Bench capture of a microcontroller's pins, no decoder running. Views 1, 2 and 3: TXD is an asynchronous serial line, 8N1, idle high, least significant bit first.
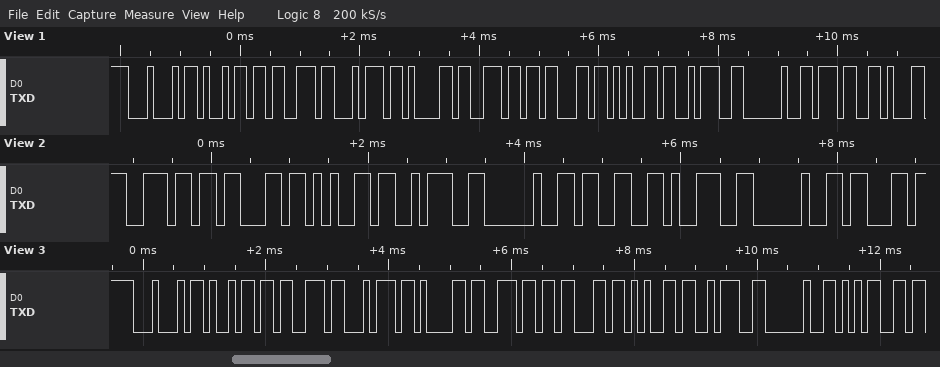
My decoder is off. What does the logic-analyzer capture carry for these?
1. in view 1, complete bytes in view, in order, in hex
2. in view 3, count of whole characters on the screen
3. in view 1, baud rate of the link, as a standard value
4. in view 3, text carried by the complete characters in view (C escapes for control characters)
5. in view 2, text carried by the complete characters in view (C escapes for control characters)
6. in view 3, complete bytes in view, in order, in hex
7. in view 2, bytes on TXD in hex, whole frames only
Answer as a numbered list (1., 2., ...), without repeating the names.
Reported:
1. 44 69 73 74 61 6E 63 65 3A 20 37
2. 11
3. 9600 baud
4. "Distance: 5"
5. "nce: 39 c"
6. 44 69 73 74 61 6E 63 65 3A 20 35
7. 6E 63 65 3A 20 33 39 20 63
